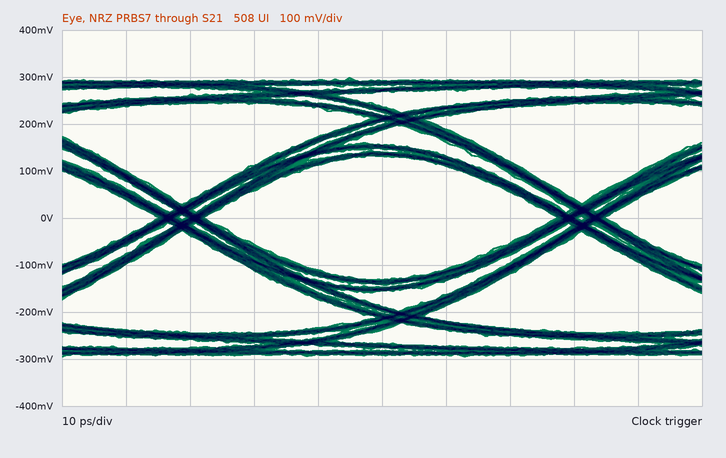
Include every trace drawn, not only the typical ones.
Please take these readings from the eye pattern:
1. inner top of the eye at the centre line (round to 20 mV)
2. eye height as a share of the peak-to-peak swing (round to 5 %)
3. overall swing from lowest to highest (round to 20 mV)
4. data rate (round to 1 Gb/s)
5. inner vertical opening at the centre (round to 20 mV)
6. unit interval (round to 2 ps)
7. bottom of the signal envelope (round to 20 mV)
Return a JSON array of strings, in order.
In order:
["140 mV", "45 %", "600 mV", "16 Gb/s", "260 mV", "62 ps", "-300 mV"]
